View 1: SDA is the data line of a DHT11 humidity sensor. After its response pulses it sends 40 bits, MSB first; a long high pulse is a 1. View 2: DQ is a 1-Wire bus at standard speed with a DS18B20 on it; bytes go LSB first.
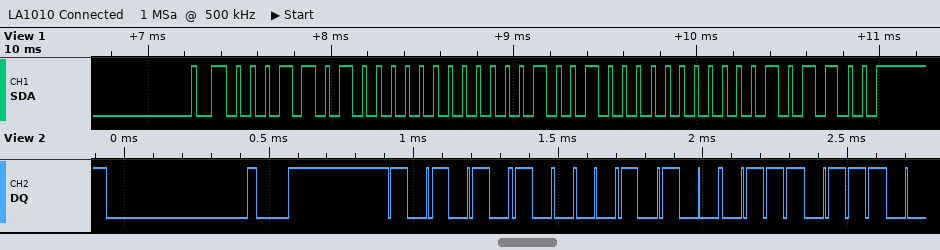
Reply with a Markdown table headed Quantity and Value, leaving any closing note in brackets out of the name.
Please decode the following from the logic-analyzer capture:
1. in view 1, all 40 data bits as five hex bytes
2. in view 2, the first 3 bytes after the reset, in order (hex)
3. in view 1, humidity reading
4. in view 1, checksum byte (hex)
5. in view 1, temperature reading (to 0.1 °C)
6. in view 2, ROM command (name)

| Quantity | Value |
|---|---|
| in view 1, all 40 data bits as five hex bytes | 1A 00 12 00 2C |
| in view 2, the first 3 bytes after the reset, in order | 55 28 EE |
| in view 1, humidity reading | 26 % |
| in view 1, checksum byte | 0x2C |
| in view 1, temperature reading | 18.0 °C |
| in view 2, ROM command | Match ROM |
